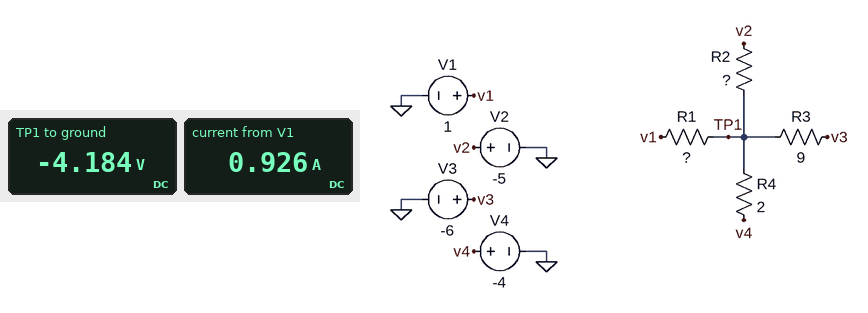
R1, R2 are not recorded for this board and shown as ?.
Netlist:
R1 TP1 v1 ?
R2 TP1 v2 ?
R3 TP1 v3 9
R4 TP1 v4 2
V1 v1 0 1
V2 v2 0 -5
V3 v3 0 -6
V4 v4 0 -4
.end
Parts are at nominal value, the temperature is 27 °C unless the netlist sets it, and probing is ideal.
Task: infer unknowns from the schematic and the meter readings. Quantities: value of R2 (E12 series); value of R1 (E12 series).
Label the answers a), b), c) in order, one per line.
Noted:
a) 1 Ω
b) 5.6 Ω
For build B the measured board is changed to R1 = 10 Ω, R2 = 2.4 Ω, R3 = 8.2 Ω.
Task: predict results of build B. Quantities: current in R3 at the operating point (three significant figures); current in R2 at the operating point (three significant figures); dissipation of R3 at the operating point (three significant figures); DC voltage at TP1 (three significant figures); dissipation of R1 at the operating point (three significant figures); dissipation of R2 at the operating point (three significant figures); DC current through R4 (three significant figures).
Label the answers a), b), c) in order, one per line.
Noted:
a) 227 mA
b) 358 mA
c) 421 mW
d) -4.14 V
e) 2.64 W
f) 307 mW
g) 70.5 mA
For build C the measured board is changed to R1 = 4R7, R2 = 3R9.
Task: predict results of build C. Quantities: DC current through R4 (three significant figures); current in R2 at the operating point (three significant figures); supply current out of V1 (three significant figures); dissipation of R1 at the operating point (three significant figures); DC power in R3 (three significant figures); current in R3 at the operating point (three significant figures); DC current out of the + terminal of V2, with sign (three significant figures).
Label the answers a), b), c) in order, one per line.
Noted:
a) 271 mA
b) 395 mA
c) 949 mA
d) 4.23 W
e) 718 mW
f) 282 mA
g) -395 mA
